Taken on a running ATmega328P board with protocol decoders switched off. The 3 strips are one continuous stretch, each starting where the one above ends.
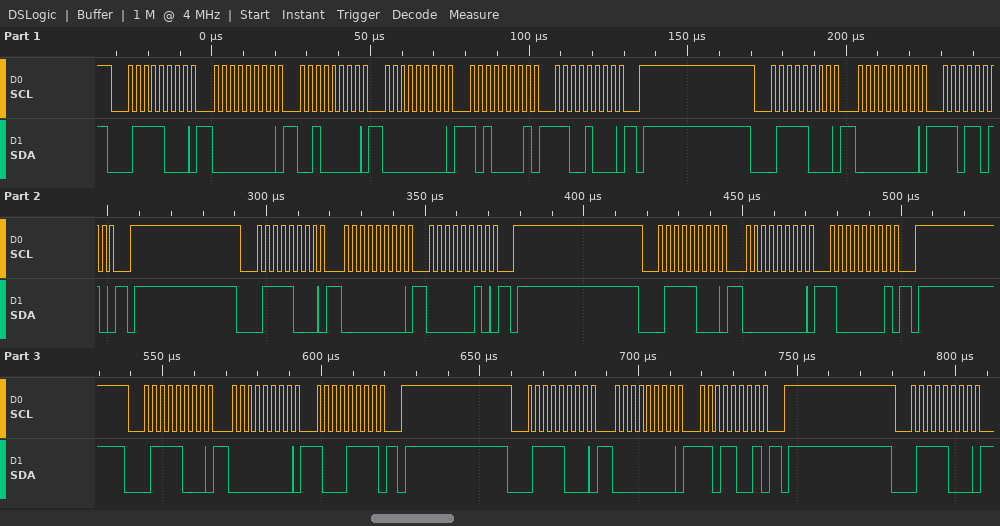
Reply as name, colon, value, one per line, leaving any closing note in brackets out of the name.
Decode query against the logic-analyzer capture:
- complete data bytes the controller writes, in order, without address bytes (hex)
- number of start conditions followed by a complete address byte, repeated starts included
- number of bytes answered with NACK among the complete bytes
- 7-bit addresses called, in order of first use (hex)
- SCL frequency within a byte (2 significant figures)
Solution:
complete data bytes the controller writes, in order, without address bytes: 00 20 00 A1 C8 00 DA 00 02 00 81 00 8F 00 D9
number of start conditions followed by a complete address byte, repeated starts included: 7
number of bytes answered with NACK among the complete bytes: 0
7-bit addresses called, in order of first use: 0x3C
SCL frequency within a byte: 400 kHz
